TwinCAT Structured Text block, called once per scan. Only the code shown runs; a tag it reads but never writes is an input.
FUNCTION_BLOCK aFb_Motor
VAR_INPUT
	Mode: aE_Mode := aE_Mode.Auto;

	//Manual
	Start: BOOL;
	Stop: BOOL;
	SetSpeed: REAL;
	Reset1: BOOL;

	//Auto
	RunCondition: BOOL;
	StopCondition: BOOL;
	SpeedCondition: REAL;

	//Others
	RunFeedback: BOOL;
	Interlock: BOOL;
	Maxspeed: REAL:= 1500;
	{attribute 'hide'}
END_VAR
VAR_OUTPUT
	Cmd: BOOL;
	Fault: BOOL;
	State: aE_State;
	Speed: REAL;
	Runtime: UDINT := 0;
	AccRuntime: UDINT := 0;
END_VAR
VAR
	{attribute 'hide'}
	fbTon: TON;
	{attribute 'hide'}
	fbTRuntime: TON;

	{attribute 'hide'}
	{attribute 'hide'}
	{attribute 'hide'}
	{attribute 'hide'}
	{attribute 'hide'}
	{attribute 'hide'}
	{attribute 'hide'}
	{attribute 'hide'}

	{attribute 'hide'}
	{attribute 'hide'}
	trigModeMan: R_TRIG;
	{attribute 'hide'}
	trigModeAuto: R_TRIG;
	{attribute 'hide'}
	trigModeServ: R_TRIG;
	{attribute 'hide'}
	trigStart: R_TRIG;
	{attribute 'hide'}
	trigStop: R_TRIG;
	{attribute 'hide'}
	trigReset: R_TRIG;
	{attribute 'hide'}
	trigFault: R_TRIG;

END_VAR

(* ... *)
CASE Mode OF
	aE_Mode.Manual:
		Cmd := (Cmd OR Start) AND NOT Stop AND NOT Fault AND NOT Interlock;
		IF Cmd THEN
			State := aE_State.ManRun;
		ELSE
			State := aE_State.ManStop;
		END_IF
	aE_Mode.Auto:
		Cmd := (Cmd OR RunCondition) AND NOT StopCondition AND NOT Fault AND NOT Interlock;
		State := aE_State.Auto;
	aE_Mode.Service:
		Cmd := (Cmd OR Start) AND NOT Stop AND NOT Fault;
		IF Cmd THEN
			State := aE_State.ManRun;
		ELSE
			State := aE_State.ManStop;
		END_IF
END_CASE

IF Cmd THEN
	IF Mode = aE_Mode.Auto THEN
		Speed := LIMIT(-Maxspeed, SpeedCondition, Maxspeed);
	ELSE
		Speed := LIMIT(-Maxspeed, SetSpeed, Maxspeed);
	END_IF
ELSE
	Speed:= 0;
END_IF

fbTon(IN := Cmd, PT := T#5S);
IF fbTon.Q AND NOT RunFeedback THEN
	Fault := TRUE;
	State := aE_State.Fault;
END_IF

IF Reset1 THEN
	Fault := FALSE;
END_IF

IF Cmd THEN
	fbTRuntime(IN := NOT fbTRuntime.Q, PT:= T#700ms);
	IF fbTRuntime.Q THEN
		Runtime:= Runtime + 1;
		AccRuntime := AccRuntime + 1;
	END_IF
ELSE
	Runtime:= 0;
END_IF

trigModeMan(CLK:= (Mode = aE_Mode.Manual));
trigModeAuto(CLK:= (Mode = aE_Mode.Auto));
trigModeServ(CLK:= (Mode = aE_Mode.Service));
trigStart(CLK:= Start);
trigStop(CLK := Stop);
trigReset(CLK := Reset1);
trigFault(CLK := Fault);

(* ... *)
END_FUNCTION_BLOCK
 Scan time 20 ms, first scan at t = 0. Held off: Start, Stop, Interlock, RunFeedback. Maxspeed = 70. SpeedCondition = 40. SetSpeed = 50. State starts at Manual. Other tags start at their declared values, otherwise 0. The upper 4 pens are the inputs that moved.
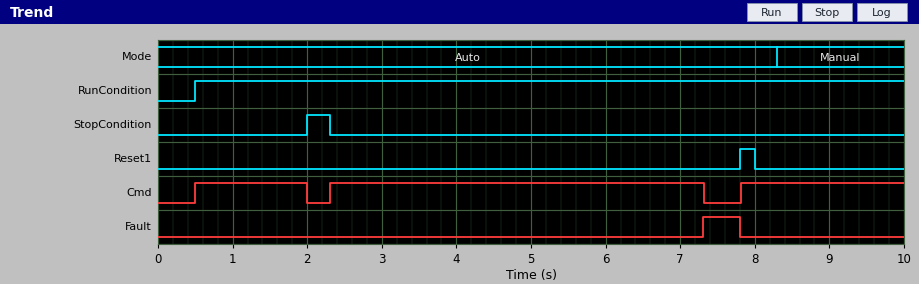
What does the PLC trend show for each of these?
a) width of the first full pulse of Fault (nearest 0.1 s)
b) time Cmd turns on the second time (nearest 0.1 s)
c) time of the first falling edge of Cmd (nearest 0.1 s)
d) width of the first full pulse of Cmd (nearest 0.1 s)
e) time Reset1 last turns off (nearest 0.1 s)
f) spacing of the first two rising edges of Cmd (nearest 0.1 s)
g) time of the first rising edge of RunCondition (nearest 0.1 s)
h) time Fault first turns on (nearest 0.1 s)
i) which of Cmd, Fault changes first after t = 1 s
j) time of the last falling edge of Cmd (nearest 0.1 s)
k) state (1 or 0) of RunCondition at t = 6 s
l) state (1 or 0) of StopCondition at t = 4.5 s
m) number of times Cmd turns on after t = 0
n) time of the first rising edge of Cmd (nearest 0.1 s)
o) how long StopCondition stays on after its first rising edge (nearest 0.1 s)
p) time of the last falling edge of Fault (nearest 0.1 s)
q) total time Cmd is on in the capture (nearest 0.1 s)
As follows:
0.5 s
2.3 s
2.0 s
1.5 s
8.0 s
1.8 s
0.5 s
7.3 s
Cmd
7.3 s
1
0
3
0.5 s
0.3 s
7.8 s
8.7 s
